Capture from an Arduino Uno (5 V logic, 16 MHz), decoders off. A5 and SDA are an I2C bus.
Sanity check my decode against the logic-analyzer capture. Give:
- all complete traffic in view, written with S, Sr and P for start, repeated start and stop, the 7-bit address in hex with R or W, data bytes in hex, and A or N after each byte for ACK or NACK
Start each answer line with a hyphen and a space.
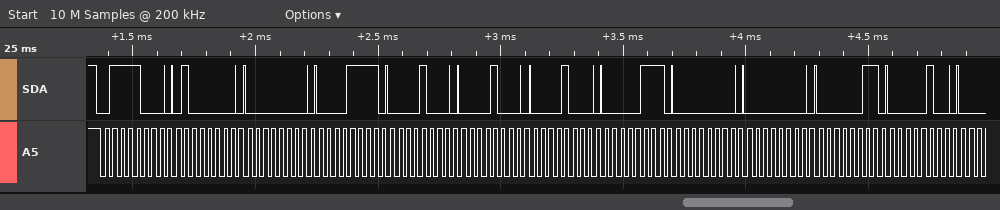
- S 3CW A 40 A 00 A 0F A 08 A 08 A 08 A 07 A 00 A 00 A 03 A 04 A
